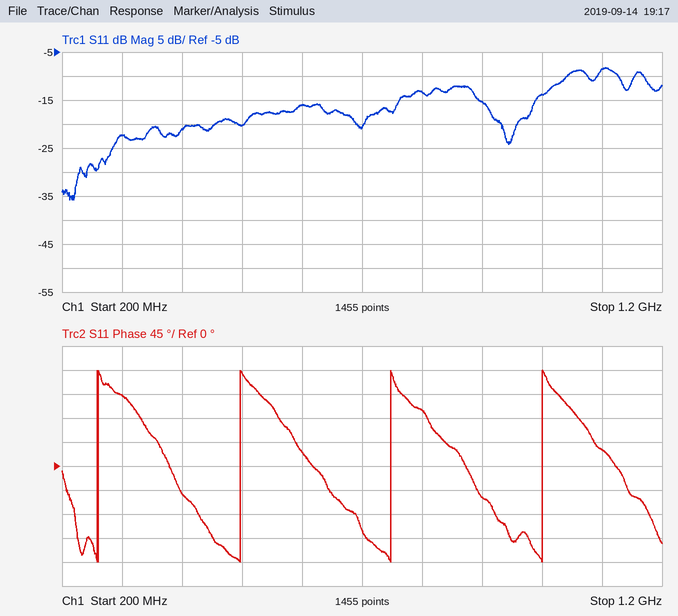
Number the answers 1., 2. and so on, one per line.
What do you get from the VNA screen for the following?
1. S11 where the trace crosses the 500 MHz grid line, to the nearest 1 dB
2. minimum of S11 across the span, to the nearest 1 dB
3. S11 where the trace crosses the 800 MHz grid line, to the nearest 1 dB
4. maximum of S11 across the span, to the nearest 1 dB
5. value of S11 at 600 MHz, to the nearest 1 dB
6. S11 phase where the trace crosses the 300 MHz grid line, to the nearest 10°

1. -20 dB
2. -36 dB
3. -13 dB
4. -8 dB
5. -16 dB
6. 130°
